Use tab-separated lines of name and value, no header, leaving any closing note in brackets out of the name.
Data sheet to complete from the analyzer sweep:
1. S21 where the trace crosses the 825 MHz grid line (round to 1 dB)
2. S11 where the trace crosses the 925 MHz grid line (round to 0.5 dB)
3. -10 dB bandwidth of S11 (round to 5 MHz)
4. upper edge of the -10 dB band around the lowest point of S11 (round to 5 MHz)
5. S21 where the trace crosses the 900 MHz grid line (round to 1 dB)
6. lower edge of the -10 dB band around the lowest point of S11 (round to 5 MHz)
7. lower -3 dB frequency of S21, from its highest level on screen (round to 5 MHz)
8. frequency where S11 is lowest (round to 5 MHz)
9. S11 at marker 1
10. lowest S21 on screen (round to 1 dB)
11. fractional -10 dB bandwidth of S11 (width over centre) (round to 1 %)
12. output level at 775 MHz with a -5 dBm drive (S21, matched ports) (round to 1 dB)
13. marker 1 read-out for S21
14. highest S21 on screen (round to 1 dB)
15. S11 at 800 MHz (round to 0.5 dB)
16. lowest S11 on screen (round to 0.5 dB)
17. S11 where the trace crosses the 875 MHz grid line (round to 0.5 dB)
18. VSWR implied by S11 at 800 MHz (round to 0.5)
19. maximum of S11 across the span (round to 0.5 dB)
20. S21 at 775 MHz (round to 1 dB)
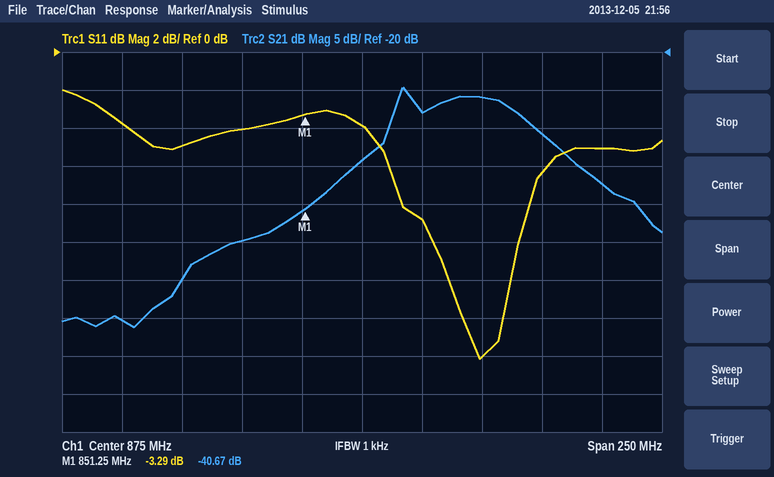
S21 where the trace crosses the 825 MHz grid line	-45 dB
S11 where the trace crosses the 925 MHz grid line	-16.0 dB
-10 dB bandwidth of S11	35 MHz
upper edge of the -10 dB band around the lowest point of S11	940 MHz
S21 where the trace crosses the 900 MHz grid line	-28 dB
lower edge of the -10 dB band around the lowest point of S11	905 MHz
lower -3 dB frequency of S21, from its highest level on screen	890 MHz
frequency where S11 is lowest	925 MHz
S11 at marker 1	-3.29 dB
lowest S21 on screen	-56 dB
fractional -10 dB bandwidth of S11 (width over centre)	4 %
output level at 775 MHz with a -5 dBm drive (S21, matched ports)	-60 dBm
marker 1 read-out for S21	-40.67 dB
highest S21 on screen	-25 dB
S11 at 800 MHz	-5.0 dB
lowest S11 on screen	-16.0 dB
S11 where the trace crosses the 875 MHz grid line	-4.0 dB
VSWR implied by S11 at 800 MHz	3.5
maximum of S11 across the span	-2.0 dB
S21 at 775 MHz	-55 dB
